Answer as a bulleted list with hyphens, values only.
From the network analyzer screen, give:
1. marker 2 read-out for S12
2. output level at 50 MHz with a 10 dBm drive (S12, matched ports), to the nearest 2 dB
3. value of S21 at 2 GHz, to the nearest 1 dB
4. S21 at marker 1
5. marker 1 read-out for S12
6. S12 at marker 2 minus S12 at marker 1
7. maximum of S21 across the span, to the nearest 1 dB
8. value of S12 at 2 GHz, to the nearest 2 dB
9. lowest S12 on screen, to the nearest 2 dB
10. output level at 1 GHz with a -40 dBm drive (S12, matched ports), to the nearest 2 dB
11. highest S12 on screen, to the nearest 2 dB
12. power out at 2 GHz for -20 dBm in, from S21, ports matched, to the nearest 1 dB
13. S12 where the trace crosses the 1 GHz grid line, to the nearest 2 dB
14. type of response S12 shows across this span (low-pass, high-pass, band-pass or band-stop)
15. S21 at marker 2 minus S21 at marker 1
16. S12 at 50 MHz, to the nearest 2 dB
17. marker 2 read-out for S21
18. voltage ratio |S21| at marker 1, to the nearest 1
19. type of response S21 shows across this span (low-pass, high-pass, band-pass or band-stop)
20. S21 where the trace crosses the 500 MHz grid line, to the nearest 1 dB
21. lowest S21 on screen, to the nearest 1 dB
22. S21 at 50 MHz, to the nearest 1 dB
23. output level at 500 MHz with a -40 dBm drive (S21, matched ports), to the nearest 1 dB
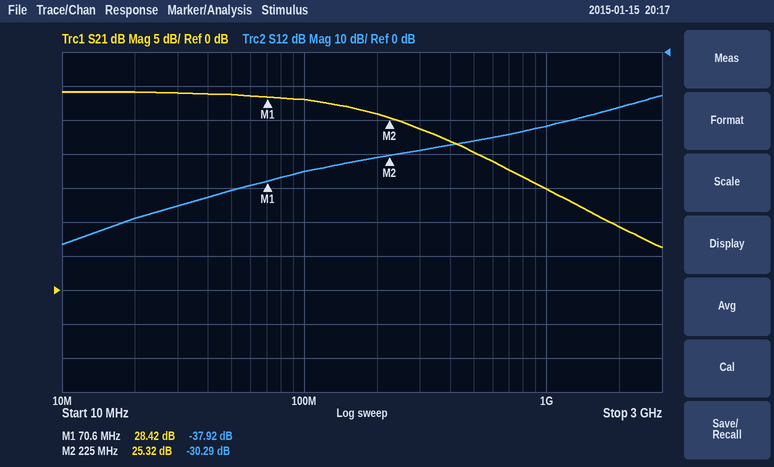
- -30.29 dB
- -30 dBm
- 9 dB
- 28.42 dB
- -37.92 dB
- 7.63 dB
- 29 dB
- -16 dB
- -56 dB
- -62 dBm
- -12 dB
- -11 dBm
- -22 dB
- high-pass
- -3.10 dB
- -40 dB
- 25.32 dB
- 26
- low-pass
- 20 dB
- 6 dB
- 29 dB
- -20 dBm
